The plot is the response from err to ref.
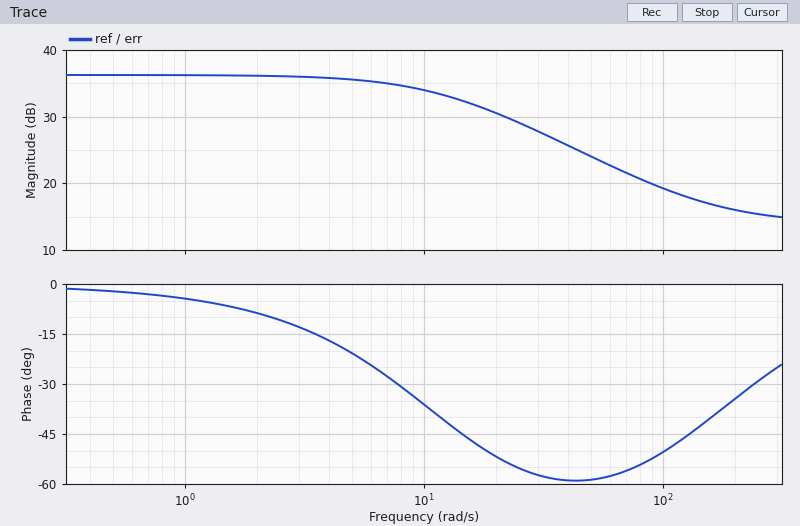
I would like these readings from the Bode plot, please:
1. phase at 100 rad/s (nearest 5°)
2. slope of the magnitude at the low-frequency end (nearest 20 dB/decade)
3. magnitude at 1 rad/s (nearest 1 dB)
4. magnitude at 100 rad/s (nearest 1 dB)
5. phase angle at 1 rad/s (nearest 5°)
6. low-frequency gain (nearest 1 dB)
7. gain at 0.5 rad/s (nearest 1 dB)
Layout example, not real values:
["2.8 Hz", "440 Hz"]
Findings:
["-50°", "0 dB/decade", "36 dB", "19 dB", "-5°", "36 dB", "36 dB"]
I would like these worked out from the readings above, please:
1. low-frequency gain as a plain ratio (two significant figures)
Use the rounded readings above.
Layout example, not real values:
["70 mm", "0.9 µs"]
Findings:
["63"]
